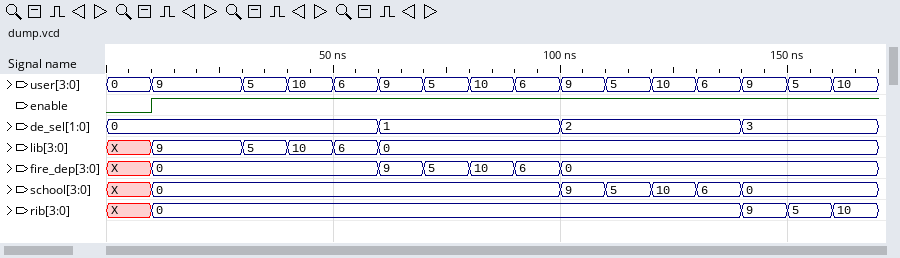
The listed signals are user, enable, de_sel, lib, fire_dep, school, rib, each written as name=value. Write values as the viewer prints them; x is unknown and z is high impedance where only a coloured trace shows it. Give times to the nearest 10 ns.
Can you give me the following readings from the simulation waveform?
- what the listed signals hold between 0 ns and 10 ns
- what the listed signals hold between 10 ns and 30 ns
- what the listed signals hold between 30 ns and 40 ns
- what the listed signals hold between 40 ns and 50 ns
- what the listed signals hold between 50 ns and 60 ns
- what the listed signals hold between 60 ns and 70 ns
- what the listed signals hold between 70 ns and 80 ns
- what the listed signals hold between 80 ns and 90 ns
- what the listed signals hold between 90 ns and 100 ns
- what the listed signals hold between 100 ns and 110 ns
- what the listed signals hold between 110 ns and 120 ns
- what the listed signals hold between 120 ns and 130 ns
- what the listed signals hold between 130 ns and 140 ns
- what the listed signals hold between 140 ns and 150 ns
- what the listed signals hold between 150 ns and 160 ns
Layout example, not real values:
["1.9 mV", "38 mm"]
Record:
["user=0, enable=0, de_sel=0, lib=X, fire_dep=X, school=X, rib=X", "user=9, enable=1, de_sel=0, lib=9, fire_dep=0, school=0, rib=0", "user=5, enable=1, de_sel=0, lib=5, fire_dep=0, school=0, rib=0", "user=10, enable=1, de_sel=0, lib=10, fire_dep=0, school=0, rib=0", "user=6, enable=1, de_sel=0, lib=6, fire_dep=0, school=0, rib=0", "user=9, enable=1, de_sel=1, lib=0, fire_dep=9, school=0, rib=0", "user=5, enable=1, de_sel=1, lib=0, fire_dep=5, school=0, rib=0", "user=10, enable=1, de_sel=1, lib=0, fire_dep=10, school=0, rib=0", "user=6, enable=1, de_sel=1, lib=0, fire_dep=6, school=0, rib=0", "user=9, enable=1, de_sel=2, lib=0, fire_dep=0, school=9, rib=0", "user=5, enable=1, de_sel=2, lib=0, fire_dep=0, school=5, rib=0", "user=10, enable=1, de_sel=2, lib=0, fire_dep=0, school=10, rib=0", "user=6, enable=1, de_sel=2, lib=0, fire_dep=0, school=6, rib=0", "user=9, enable=1, de_sel=3, lib=0, fire_dep=0, school=0, rib=9", "user=5, enable=1, de_sel=3, lib=0, fire_dep=0, school=0, rib=5"]
